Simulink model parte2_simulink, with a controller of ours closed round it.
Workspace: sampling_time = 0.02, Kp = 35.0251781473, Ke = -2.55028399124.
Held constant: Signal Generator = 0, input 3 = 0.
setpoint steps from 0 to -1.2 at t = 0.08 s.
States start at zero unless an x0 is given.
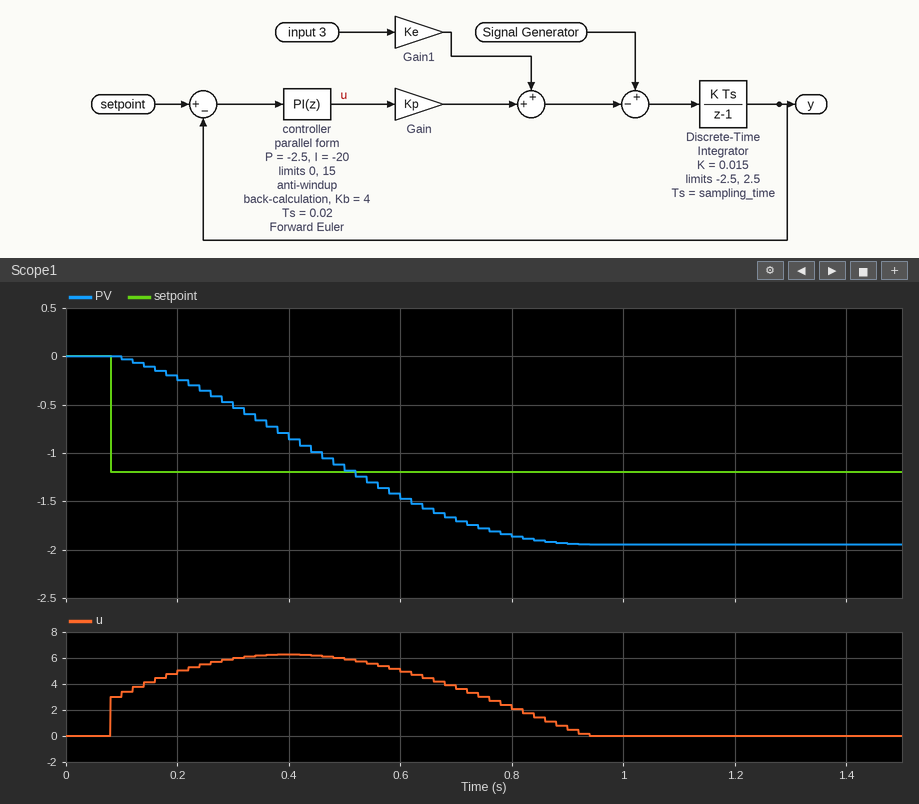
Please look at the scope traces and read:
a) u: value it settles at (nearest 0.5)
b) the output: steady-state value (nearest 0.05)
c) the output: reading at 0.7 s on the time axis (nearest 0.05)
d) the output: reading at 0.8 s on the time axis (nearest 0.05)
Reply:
0.0
-1.95
-1.70
-1.85
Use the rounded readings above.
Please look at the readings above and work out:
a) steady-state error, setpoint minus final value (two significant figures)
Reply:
0.75
